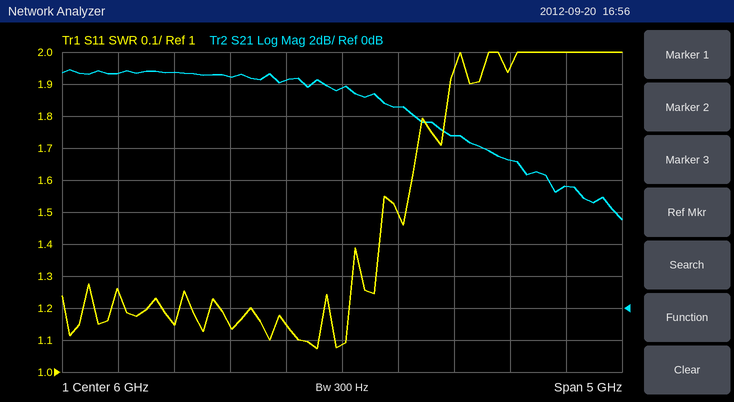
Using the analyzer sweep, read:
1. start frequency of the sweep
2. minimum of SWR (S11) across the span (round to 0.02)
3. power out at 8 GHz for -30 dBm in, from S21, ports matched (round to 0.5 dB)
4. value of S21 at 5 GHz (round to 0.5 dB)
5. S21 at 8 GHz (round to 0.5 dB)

3.5 GHz
1.08
-22.5 dBm
14.5 dB
7.5 dB
